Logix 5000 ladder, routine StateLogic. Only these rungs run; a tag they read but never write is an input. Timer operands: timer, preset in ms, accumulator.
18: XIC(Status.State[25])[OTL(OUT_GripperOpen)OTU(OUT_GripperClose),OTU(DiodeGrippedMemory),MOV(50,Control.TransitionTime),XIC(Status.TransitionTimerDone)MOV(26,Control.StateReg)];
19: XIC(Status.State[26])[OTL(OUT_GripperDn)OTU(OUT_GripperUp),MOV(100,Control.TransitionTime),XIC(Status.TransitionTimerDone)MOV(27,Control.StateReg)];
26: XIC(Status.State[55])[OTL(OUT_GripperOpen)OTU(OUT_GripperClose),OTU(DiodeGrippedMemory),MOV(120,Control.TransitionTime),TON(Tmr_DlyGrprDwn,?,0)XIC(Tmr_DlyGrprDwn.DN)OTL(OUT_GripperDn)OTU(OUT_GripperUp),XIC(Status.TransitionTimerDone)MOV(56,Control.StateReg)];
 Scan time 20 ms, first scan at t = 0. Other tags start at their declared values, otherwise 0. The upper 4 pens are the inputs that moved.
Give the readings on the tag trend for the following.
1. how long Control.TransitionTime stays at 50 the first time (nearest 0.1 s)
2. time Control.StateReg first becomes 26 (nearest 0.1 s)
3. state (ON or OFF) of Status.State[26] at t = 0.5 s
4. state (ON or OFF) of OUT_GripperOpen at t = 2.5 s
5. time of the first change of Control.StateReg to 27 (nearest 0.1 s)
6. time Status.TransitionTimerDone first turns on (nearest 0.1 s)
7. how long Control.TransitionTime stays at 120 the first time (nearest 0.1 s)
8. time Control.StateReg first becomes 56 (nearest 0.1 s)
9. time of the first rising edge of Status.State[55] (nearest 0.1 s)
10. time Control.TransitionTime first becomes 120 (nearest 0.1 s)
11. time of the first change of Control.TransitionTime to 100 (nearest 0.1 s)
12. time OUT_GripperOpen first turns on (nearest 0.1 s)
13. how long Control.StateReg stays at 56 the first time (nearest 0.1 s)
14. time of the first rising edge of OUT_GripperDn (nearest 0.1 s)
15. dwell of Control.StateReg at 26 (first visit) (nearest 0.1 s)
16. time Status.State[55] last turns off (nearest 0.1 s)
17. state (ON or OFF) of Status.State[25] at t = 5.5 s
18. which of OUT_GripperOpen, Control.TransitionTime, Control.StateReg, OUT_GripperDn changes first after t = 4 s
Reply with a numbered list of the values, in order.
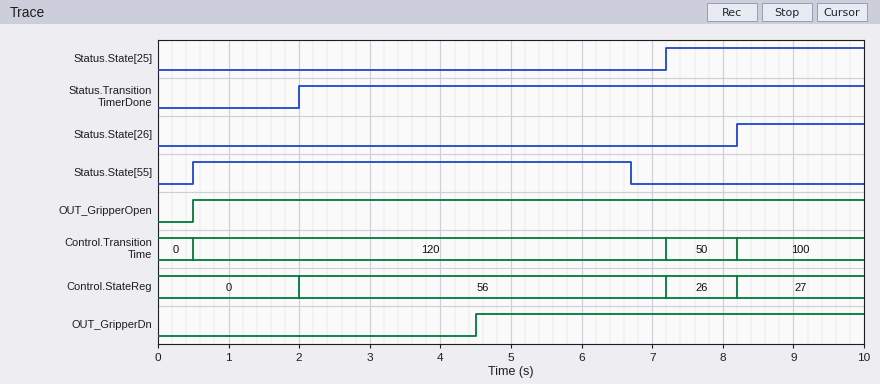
1. 1.0 s
2. 7.2 s
3. OFF
4. ON
5. 8.2 s
6. 2.0 s
7. 6.7 s
8. 2.0 s
9. 0.5 s
10. 0.5 s
11. 8.2 s
12. 0.5 s
13. 5.2 s
14. 4.5 s
15. 1.0 s
16. 6.7 s
17. OFF
18. OUT_GripperDn
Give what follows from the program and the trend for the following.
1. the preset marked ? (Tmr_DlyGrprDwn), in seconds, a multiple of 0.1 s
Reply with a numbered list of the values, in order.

1. 4.0 s
